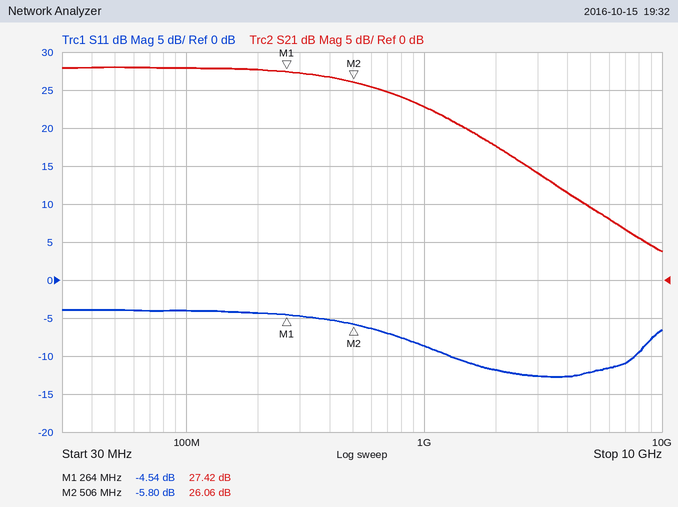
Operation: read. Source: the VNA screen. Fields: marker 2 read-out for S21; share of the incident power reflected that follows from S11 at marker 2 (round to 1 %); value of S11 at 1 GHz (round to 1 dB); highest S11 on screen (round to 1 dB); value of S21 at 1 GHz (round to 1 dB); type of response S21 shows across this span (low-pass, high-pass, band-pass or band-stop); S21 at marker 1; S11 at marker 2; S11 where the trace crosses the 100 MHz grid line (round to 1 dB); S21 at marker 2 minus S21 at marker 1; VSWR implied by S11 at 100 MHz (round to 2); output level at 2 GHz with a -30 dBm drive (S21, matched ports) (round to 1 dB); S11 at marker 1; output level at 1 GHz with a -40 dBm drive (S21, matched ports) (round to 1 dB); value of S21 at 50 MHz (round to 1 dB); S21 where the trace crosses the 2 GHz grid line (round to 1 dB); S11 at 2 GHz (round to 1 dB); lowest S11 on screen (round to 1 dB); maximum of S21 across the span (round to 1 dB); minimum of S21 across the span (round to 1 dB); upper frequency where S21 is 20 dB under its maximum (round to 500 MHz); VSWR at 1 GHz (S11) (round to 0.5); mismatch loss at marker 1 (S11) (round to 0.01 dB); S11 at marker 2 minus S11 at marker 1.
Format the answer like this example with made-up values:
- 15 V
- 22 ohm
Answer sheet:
- 26.06 dB
- 26 %
- -9 dB
- -4 dB
- 23 dB
- low-pass
- 27.42 dB
- -5.80 dB
- -4 dB
- -1.36 dB
- 4
- -12 dBm
- -4.54 dB
- -17 dBm
- 28 dB
- 18 dB
- -12 dB
- -13 dB
- 28 dB
- 4 dB
- 6.0 GHz
- 2.0
- 1.88 dB
- -1.26 dB
